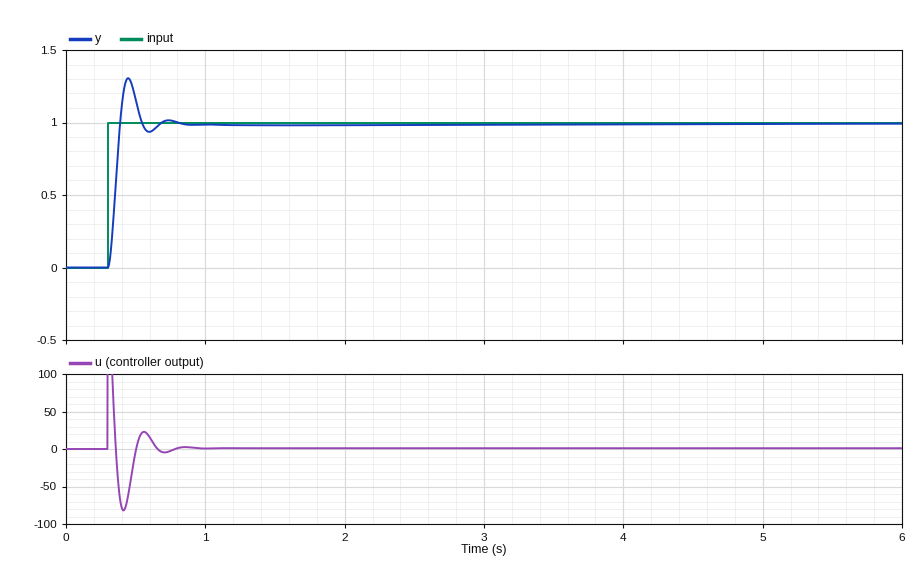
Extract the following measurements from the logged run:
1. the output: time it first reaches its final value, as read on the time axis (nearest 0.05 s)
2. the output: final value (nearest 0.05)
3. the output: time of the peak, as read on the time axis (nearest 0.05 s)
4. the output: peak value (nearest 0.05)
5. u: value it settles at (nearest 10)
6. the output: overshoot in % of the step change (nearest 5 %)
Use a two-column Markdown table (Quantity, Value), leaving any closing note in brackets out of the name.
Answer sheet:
| Quantity | Value |
|---|---|
| the output: time it first reaches its final value, as read on the time axis | 0.40 s |
| the output: final value | 1.00 |
| the output: time of the peak, as read on the time axis | 0.45 s |
| the output: peak value | 1.30 |
| u: value it settles at | 0 |
| the output: overshoot in % of the step change | 30 % |
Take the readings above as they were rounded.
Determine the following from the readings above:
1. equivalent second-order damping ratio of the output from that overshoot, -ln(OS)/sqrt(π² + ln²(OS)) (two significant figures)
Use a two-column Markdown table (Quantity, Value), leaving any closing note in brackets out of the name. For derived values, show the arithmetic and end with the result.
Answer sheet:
| Quantity | Value |
|---|---|
| equivalent second-order damping ratio of the output from that overshoot, -ln(OS)/sqrt(π² + ln²(OS)) | ln(0.3) = -1.204; 1.204 / sqrt(9.870 + 1.450) = 0.36 |
